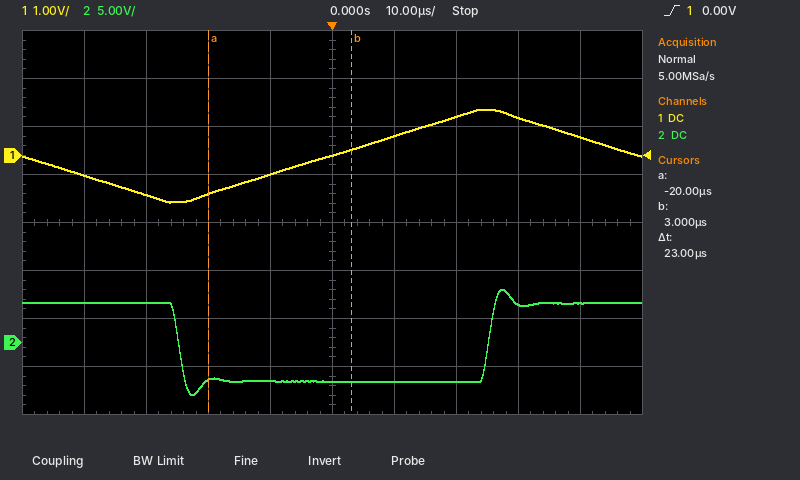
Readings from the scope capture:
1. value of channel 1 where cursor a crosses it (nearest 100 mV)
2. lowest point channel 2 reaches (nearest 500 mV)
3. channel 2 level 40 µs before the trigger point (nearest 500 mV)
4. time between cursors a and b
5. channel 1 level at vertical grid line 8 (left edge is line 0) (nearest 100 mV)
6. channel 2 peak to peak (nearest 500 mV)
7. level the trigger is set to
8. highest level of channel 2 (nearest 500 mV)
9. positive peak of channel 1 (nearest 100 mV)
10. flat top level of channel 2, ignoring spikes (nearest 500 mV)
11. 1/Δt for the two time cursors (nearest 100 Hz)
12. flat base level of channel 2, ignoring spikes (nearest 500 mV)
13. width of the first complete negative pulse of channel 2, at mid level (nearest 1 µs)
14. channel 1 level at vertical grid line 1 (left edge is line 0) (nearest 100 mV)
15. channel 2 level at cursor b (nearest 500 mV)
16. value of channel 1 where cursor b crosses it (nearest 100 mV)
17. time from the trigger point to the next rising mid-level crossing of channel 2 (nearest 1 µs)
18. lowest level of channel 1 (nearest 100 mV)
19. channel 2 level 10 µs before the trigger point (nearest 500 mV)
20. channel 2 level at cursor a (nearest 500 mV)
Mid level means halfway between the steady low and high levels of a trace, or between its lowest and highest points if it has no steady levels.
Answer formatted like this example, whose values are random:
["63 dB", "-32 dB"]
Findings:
["-800 mV", "-5.5 V", "4.0 V", "23 µs", "800 mV", "11.0 V", "0.00 V", "5.5 V", "1.0 V", "4.0 V", "43.5 kHz", "-4.0 V", "50 µs", "-400 mV", "-4.0 V", "100 mV", "25 µs", "-1.0 V", "-4.0 V", "-4.0 V"]
